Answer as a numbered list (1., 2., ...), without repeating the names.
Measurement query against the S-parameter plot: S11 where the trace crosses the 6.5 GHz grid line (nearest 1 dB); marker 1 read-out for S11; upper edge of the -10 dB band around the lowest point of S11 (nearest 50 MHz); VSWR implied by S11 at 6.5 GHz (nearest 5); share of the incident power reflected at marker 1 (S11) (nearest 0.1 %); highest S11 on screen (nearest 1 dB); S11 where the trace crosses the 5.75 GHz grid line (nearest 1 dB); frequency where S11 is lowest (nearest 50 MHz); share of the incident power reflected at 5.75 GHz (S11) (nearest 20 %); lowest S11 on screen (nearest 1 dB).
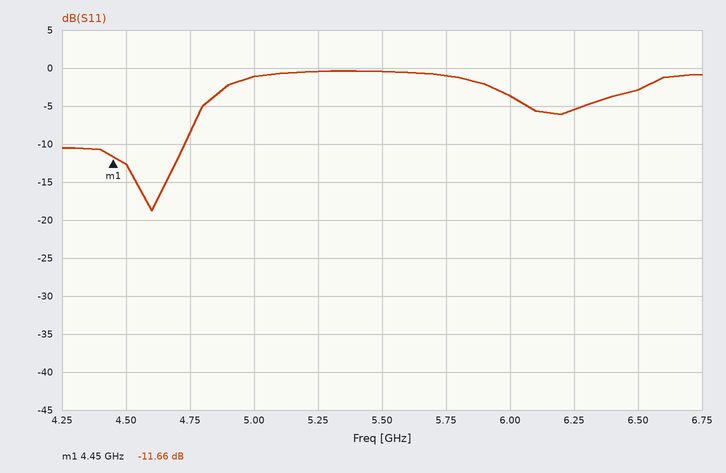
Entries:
1. -3 dB
2. -11.66 dB
3. 4.75 GHz
4. 5
5. 6.8 %
6. 0 dB
7. -1 dB
8. 4.60 GHz
9. 80 %
10. -19 dB
